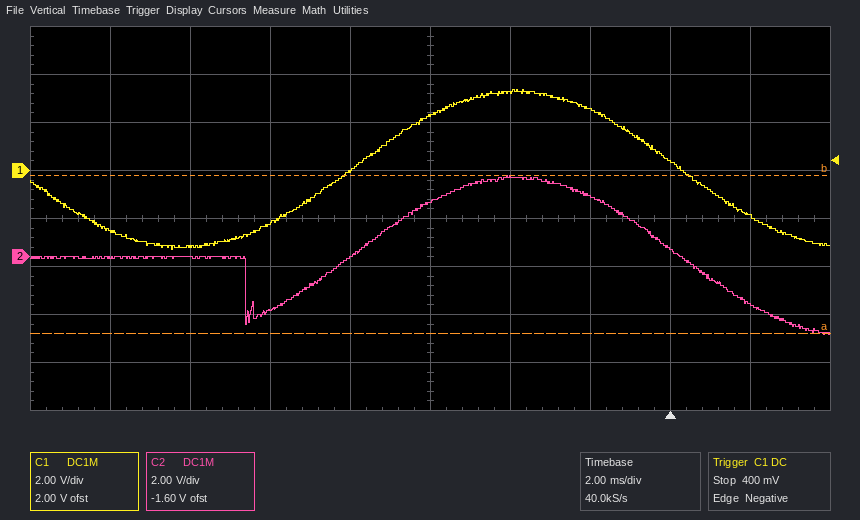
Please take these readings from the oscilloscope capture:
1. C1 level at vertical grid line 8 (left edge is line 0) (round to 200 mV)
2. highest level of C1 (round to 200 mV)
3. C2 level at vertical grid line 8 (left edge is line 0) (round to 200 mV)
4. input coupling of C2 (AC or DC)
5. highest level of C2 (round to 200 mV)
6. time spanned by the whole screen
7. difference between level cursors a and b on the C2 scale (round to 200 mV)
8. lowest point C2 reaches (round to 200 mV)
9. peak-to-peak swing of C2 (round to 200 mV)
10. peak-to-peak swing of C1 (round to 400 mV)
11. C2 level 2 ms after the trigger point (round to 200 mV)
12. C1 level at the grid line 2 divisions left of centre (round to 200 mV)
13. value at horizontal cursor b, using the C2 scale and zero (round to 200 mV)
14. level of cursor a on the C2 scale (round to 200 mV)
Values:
400 mV
3.4 V
400 mV
DC
3.4 V
20 ms
6.6 V
-3.2 V
6.6 V
6.8 V
-2.0 V
-2.2 V
3.4 V
-3.2 V
